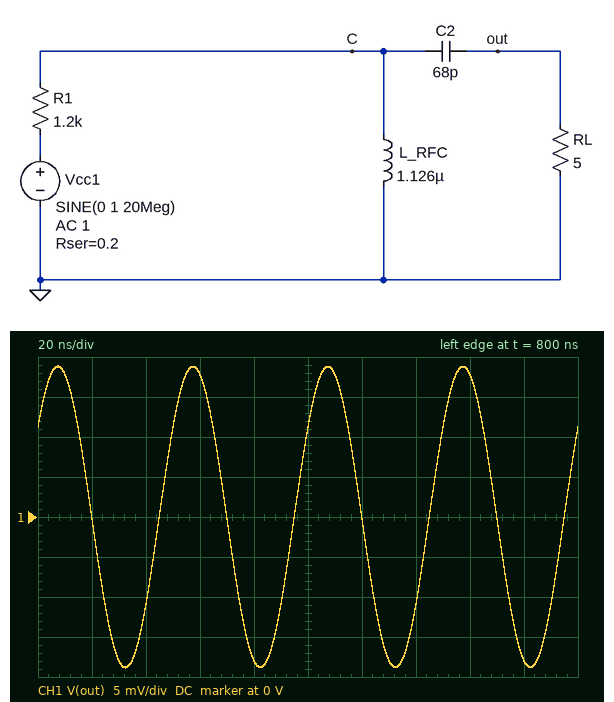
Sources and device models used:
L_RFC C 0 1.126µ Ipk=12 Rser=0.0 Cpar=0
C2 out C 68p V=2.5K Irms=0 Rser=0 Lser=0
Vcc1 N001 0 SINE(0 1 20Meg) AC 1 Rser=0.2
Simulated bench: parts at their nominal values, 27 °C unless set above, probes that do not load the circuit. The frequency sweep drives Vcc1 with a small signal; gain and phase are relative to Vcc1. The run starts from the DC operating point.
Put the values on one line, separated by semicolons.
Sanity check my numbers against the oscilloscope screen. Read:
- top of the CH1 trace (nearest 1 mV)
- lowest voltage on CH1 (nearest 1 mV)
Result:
19 mV; -19 mV
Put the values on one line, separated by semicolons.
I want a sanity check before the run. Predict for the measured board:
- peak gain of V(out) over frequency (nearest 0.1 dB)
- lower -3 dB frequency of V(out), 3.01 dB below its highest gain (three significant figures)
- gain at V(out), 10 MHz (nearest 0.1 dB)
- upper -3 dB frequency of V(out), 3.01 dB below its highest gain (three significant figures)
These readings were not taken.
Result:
-30.9 dB; 17.0 MHz; -54.9 dB; 19.8 MHz
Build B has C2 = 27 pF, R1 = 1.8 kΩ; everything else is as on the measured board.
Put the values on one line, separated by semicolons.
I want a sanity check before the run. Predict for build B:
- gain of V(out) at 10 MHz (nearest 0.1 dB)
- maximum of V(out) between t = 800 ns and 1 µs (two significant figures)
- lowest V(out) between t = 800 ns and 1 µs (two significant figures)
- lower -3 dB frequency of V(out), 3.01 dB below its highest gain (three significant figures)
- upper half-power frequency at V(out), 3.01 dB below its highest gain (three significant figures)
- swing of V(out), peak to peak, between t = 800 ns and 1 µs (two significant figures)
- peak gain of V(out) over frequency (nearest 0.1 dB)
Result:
-68.4 dB; 2.5 mV; -2.5 mV; 27.1 MHz; 31.2 MHz; 5.1 mV; -33.9 dB
